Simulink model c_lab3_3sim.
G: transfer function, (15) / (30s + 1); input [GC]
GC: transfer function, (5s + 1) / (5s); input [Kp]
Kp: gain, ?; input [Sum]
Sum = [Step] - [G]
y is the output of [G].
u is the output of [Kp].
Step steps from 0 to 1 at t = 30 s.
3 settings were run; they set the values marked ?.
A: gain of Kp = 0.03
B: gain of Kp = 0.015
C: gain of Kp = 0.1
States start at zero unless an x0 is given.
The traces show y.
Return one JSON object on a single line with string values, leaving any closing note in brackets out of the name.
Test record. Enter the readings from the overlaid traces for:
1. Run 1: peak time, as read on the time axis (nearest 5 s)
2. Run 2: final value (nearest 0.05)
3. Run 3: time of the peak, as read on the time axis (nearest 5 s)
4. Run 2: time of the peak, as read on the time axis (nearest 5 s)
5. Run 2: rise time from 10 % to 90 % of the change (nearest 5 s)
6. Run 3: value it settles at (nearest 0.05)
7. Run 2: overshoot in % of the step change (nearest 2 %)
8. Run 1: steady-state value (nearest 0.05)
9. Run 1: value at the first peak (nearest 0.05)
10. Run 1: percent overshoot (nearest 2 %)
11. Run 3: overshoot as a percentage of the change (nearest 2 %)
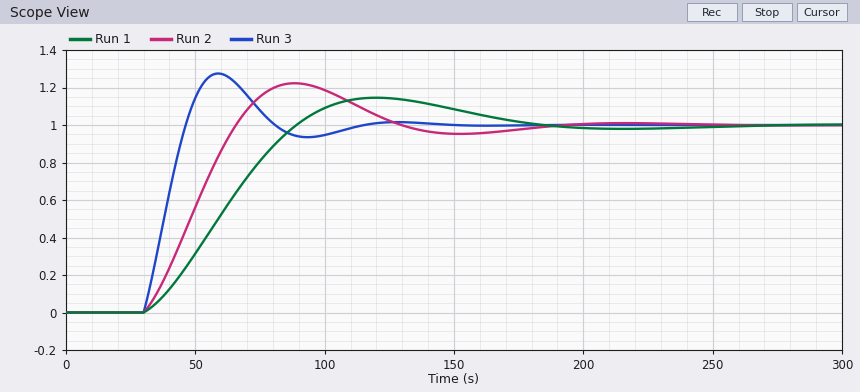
{"Run 1: peak time, as read on the time axis": "120 s", "Run 2: final value": "1.00", "Run 3: time of the peak, as read on the time axis": "60 s", "Run 2: time of the peak, as read on the time axis": "90 s", "Run 2: rise time from 10 % to 90 % of the change": "25 s", "Run 3: value it settles at": "1.00", "Run 2: overshoot in % of the step change": "22 %", "Run 1: steady-state value": "1.00", "Run 1: value at the first peak": "1.15", "Run 1: percent overshoot": "14 %", "Run 3: overshoot as a percentage of the change": "28 %"}
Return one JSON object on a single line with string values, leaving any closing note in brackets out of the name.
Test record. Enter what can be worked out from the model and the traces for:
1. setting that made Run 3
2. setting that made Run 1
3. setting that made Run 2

{"setting that made Run 3": "C", "setting that made Run 1": "B", "setting that made Run 2": "A"}
